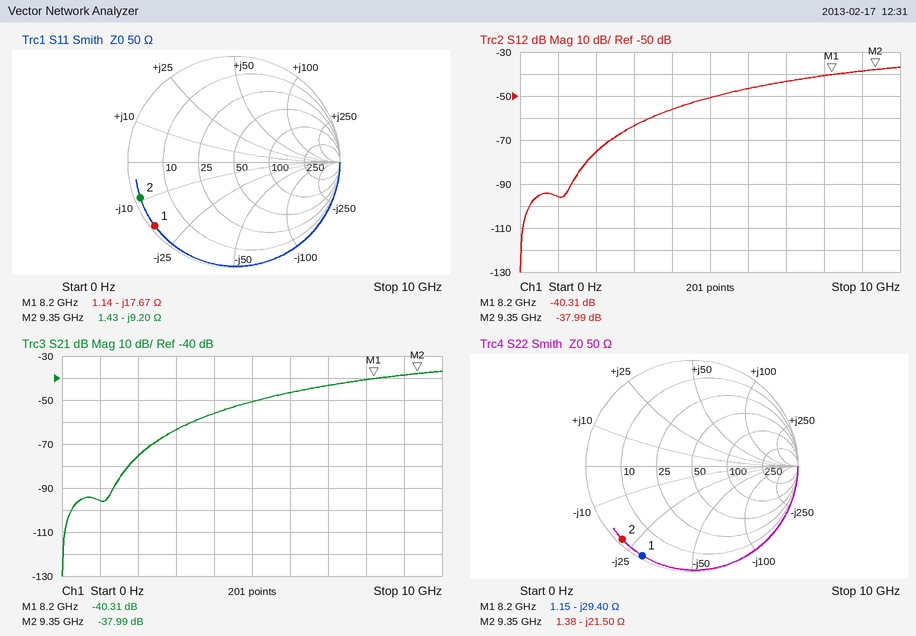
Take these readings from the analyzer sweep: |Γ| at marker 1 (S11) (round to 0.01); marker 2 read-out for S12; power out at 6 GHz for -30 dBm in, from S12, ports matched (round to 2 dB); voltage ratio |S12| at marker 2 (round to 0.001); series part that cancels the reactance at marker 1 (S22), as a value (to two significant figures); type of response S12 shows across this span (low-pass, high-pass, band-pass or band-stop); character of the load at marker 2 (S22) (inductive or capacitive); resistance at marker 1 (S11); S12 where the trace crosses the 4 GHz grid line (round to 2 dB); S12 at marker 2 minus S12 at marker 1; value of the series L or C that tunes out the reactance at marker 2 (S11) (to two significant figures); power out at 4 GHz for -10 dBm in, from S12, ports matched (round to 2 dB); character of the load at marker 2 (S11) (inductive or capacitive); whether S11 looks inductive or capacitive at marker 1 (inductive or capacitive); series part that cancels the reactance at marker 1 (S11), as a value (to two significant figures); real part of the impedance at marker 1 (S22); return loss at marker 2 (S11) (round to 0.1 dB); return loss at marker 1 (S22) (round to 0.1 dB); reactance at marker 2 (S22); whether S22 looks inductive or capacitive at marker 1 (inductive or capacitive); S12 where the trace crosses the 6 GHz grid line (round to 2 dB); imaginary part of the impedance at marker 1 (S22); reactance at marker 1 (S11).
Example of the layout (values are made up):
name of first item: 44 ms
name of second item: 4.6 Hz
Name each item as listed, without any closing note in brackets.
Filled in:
|Γ| at marker 1 (S11): 0.96
marker 2 read-out for S12: -37.99 dB
power out at 6 GHz for -30 dBm in, from S12, ports matched: -76 dBm
voltage ratio |S12| at marker 2: 0.013
series part that cancels the reactance at marker 1 (S22), as a value: 570 pH
type of response S12 shows across this span: high-pass
character of the load at marker 2 (S22): capacitive
resistance at marker 1: 1.14 Ω
S12 where the trace crosses the 4 GHz grid line: -56 dB
S12 at marker 2 minus S12 at marker 1: 2.32 dB
value of the series L or C that tunes out the reactance at marker 2 (S11): 160 pH
power out at 4 GHz for -10 dBm in, from S12, ports matched: -66 dBm
character of the load at marker 2 (S11): capacitive
whether S11 looks inductive or capacitive at marker 1: capacitive
series part that cancels the reactance at marker 1 (S11), as a value: 340 pH
real part of the impedance at marker 1: 1.15 Ω
return loss at marker 2 (S11): 0.5 dB
return loss at marker 1 (S22): 0.3 dB
reactance at marker 2: -21.50 Ω
whether S22 looks inductive or capacitive at marker 1: capacitive
S12 where the trace crosses the 6 GHz grid line: -46 dB
imaginary part of the impedance at marker 1: -29.40 Ω
reactance at marker 1: -17.67 Ω
